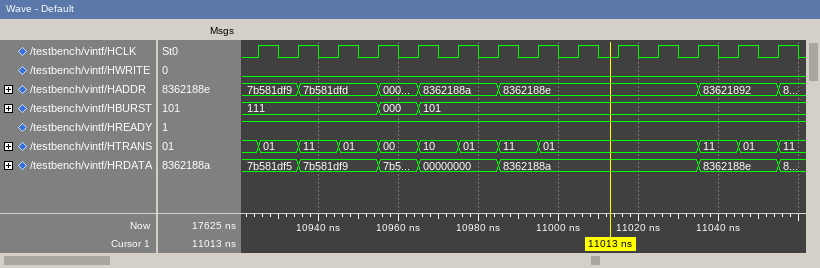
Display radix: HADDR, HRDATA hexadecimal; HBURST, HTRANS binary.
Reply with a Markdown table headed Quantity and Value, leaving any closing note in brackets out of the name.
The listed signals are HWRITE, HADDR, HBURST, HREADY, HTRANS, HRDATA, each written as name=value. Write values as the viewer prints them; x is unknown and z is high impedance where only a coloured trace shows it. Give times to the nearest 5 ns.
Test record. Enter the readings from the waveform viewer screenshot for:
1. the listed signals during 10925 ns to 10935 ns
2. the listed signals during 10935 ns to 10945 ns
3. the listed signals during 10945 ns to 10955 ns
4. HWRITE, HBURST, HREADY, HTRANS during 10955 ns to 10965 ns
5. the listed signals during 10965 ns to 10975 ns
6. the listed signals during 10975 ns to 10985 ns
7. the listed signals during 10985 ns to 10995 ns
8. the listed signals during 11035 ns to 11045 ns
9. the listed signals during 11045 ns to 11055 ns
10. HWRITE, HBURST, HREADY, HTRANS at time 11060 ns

| Quantity | Value |
|---|---|
| the listed signals during 10925 ns to 10935 ns | HWRITE=0, HADDR=7b581df9, HBURST=111, HREADY=1, HTRANS=01, HRDATA=7b581df5 |
| the listed signals during 10935 ns to 10945 ns | HWRITE=0, HADDR=7b581dfd, HBURST=111, HREADY=1, HTRANS=11, HRDATA=7b581df9 |
| the listed signals during 10945 ns to 10955 ns | HWRITE=0, HADDR=7b581dfd, HBURST=111, HREADY=1, HTRANS=01, HRDATA=7b581df9 |
| HWRITE, HBURST, HREADY, HTRANS during 10955 ns to 10965 ns | HWRITE=0, HBURST=000, HREADY=1, HTRANS=00 |
| the listed signals during 10965 ns to 10975 ns | HWRITE=0, HADDR=8362188a, HBURST=101, HREADY=1, HTRANS=10, HRDATA=00000000 |
| the listed signals during 10975 ns to 10985 ns | HWRITE=0, HADDR=8362188a, HBURST=101, HREADY=1, HTRANS=01, HRDATA=00000000 |
| the listed signals during 10985 ns to 10995 ns | HWRITE=0, HADDR=8362188e, HBURST=101, HREADY=1, HTRANS=11, HRDATA=8362188a |
| the listed signals during 11035 ns to 11045 ns | HWRITE=0, HADDR=83621892, HBURST=101, HREADY=1, HTRANS=11, HRDATA=8362188e |
| the listed signals during 11045 ns to 11055 ns | HWRITE=0, HADDR=83621892, HBURST=101, HREADY=1, HTRANS=01, HRDATA=8362188e |
| HWRITE, HBURST, HREADY, HTRANS at time 11060 ns | HWRITE=0, HBURST=101, HREADY=1, HTRANS=11 |
